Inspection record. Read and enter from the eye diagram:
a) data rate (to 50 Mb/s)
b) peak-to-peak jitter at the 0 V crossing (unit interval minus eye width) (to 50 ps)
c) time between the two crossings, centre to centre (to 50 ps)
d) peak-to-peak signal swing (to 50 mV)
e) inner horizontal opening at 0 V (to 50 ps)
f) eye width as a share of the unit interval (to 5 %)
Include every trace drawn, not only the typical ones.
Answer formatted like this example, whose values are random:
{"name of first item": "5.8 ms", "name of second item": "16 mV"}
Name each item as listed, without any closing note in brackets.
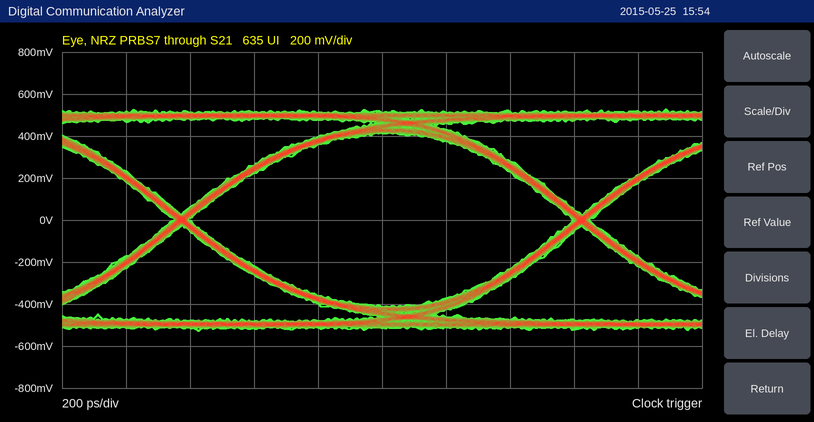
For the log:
{"data rate": "800 Mb/s", "peak-to-peak jitter at the 0 V crossing (unit interval minus eye width)": "50 ps", "time between the two crossings, centre to centre": "1.25 ns", "peak-to-peak signal swing": "1.05 V", "inner horizontal opening at 0 V": "1.20 ns", "eye width as a share of the unit interval": "95 %"}
